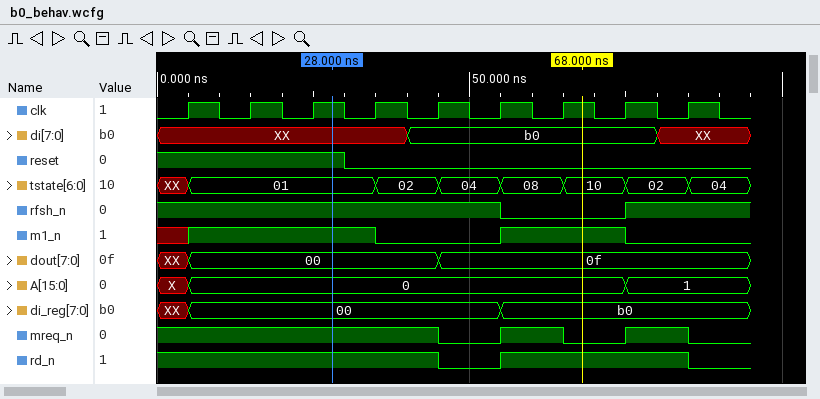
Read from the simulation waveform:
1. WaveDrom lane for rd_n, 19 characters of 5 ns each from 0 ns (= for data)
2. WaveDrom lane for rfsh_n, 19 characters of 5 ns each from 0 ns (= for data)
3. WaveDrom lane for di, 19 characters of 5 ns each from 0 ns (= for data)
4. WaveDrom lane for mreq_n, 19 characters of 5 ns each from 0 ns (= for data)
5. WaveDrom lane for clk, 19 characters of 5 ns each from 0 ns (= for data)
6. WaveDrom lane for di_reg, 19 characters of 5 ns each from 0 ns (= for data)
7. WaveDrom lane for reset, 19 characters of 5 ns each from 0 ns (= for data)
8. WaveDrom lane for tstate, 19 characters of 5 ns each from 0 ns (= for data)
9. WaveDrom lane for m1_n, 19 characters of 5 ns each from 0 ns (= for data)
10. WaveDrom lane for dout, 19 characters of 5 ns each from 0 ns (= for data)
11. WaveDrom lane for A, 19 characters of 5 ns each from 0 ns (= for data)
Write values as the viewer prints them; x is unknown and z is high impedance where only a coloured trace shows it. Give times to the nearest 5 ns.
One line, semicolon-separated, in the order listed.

{name: 'rd_n', wave: '1........0.1.....0.'}; {name: 'rfsh_n', wave: '1..........0...1...'}; {name: 'di', wave: 'x.......=.......x..', data: 'b0'}; {name: 'mreq_n', wave: '1........0.1.0.1.0.'}; {name: 'clk', wave: '0101010101010101010'}; {name: 'di_reg', wave: 'x=.........=.......', data: '00 b0'}; {name: 'reset', wave: '1.....0............'}; {name: 'tstate', wave: 'x=.....=.=.=.=.=.=.', data: '01 02 04 08 10 02 04'}; {name: 'm1_n', wave: 'x1.....0...1...0...'}; {name: 'dout', wave: 'x=.......=.........', data: '00 0f'}; {name: 'A', wave: 'x=.............=...', data: '0 1'}
